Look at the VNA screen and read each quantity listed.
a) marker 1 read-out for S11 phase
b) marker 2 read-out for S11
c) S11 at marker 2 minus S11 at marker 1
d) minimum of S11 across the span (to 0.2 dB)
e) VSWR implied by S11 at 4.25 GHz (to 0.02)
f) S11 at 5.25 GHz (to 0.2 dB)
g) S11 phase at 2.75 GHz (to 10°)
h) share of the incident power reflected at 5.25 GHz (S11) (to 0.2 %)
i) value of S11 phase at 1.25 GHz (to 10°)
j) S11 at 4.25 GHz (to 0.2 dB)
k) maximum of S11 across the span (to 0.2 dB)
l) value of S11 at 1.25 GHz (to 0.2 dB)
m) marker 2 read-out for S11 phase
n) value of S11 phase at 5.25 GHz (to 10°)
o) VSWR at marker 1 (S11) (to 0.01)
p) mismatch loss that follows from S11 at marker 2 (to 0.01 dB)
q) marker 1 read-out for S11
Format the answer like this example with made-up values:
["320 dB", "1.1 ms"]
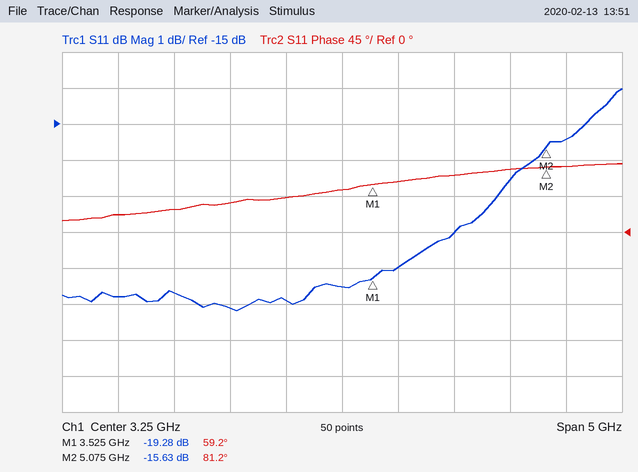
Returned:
["59.2°", "-15.63 dB", "3.65 dB", "-20.2 dB", "1.28", "-15.4 dB", "40°", "2.8 %", "20°", "-18.0 dB", "-14.0 dB", "-19.8 dB", "81.2°", "80°", "1.24", "0.12 dB", "-19.28 dB"]
